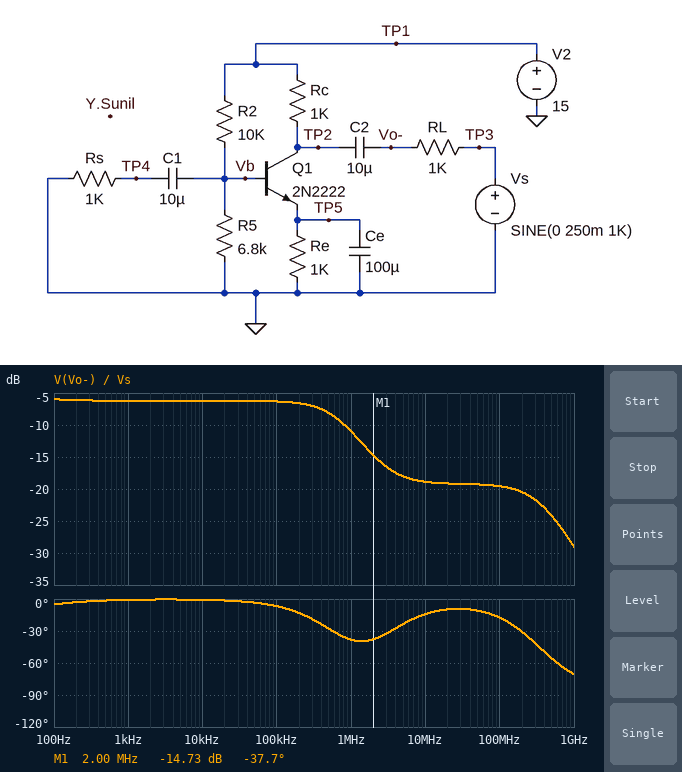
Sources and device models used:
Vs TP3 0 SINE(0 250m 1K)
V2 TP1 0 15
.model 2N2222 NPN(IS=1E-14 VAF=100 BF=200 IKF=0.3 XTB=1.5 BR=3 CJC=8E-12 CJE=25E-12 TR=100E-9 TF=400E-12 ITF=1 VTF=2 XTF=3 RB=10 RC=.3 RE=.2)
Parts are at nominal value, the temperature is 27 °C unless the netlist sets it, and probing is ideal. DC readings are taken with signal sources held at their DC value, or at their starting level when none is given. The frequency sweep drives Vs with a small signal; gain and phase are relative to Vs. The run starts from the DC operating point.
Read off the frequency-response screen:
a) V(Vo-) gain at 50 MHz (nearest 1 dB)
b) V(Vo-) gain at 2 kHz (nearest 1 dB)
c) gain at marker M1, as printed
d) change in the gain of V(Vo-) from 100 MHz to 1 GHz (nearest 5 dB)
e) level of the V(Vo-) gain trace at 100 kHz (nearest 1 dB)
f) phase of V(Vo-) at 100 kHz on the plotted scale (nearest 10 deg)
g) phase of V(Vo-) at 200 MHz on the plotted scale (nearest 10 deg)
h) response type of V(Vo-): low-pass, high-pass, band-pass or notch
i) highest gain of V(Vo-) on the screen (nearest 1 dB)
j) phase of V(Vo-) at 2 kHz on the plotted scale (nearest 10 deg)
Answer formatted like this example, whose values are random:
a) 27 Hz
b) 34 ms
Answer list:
a) -19 dB
b) -6 dB
c) -14.73 dB
d) -10 dB
e) -6 dB
f) -10 deg
g) -30 deg
h) low-pass
i) -6 dB
j) 0 deg
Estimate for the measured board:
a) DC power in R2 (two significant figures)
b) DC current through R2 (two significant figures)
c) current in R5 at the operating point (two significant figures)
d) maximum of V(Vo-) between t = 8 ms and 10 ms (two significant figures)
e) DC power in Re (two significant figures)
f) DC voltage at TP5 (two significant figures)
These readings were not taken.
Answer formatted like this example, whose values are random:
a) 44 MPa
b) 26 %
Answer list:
a) 8.2 mW
b) 900 µA
c) 880 µA
d) 120 mV
e) 28 mW
f) 5.3 V
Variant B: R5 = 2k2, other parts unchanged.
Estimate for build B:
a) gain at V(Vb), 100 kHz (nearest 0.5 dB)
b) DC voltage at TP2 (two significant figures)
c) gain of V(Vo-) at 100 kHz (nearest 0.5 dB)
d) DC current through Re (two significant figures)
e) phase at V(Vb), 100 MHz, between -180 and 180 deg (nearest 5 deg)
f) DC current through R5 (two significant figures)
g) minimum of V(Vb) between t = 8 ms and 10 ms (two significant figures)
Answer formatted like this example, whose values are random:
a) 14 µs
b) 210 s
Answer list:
a) -65.5 dB
b) 13 V
c) -6.0 dB
d) 2.0 mA
e) -20 deg
f) 1.2 mA
g) 2.7 V
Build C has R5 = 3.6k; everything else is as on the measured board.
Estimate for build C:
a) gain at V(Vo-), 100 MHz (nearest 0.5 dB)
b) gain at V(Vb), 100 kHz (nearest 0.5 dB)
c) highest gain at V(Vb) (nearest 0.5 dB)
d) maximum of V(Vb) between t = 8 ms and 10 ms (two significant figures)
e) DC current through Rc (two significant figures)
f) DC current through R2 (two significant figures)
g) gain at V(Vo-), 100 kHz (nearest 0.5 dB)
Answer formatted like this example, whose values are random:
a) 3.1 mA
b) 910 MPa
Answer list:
a) -17.0 dB
b) -65.0 dB
c) -45.0 dB
d) 3.9 V
e) 3.2 mA
f) 1.1 mA
g) -6.0 dB
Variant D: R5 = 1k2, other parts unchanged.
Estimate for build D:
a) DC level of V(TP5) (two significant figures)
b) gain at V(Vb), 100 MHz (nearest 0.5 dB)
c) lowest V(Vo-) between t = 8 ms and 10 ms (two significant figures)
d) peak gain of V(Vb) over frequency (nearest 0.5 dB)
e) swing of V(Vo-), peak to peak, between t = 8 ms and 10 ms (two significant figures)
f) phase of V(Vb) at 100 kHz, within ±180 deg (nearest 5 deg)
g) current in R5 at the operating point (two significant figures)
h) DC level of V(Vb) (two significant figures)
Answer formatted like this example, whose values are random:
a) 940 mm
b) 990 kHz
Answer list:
a) 950 mV
b) -38.5 dB
c) -120 mV
d) -37.5 dB
e) 250 mV
f) 90 deg
g) 1.3 mA
h) 1.6 V
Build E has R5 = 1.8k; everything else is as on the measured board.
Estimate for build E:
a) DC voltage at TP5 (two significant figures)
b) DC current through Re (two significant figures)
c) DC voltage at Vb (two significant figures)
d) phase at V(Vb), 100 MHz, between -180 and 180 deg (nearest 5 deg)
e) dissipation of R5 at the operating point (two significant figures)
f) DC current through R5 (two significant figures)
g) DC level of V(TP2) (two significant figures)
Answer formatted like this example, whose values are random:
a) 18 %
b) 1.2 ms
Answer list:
a) 1.6 V
b) 1.6 mA
c) 2.3 V
d) -20 deg
e) 2.9 mW
f) 1.3 mA
g) 13 V
